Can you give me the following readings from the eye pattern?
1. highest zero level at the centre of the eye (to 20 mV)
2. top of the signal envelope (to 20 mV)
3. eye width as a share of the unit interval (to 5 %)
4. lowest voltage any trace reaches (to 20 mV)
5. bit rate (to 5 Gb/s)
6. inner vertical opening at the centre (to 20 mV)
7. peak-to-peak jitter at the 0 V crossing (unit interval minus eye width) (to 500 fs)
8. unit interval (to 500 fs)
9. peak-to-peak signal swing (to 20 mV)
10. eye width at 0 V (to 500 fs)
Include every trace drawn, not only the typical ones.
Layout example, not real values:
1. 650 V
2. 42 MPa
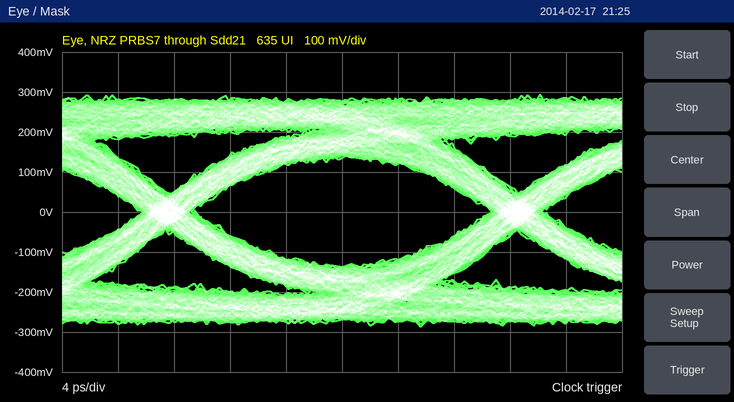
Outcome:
1. -140 mV
2. 300 mV
3. 85 %
4. -280 mV
5. 40 Gb/s
6. 280 mV
7. 4.0 ps
8. 25.0 ps
9. 580 mV
10. 21.0 ps
